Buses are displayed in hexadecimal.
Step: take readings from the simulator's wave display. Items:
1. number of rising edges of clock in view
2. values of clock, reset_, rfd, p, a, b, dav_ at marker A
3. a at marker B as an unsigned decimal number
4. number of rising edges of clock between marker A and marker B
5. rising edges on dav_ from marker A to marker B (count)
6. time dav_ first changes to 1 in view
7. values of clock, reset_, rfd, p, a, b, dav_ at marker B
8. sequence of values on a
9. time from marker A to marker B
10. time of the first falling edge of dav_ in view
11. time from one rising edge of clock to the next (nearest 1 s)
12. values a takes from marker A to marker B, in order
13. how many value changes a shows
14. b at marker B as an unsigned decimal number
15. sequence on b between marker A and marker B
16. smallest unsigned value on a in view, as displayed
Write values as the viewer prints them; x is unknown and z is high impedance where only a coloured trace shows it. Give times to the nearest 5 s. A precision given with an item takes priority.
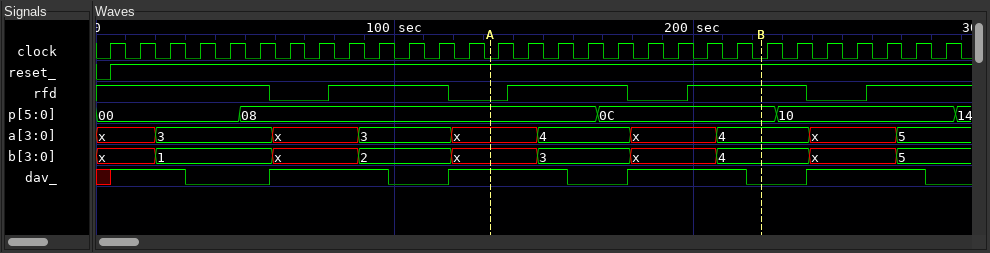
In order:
29
clock=0, reset_=1, rfd=0, p=08, a=x, b=x, dav_=1
4
9
1
5 s
clock=0, reset_=1, rfd=1, p=0C, a=4, b=4, dav_=0
x, 3, x, 3, x, 4, x, 4, x, 5
90 s
30 s
10 s
x, 4, x, 4
9
4
x, 3, x, 4
3
